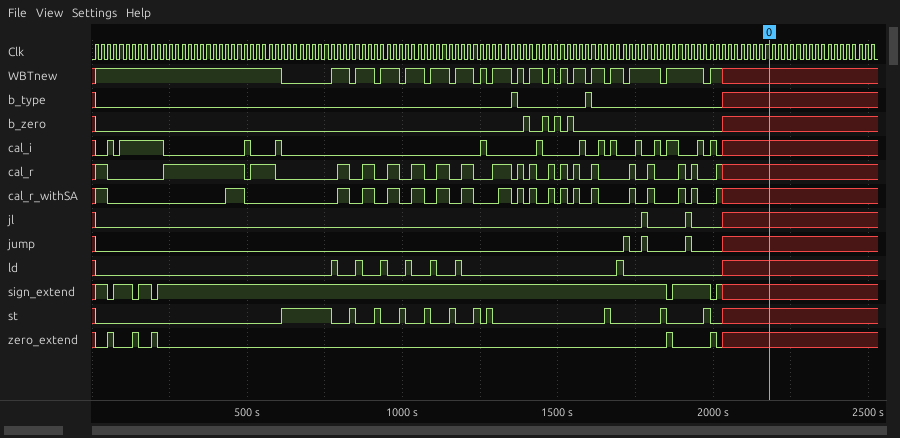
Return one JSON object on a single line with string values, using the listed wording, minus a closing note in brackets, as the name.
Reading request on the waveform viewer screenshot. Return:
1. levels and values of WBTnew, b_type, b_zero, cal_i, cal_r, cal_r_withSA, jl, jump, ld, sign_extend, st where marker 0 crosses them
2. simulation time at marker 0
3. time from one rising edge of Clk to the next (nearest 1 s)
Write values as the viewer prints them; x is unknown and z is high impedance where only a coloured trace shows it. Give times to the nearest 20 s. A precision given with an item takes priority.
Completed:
{"levels and values of WBTnew, b_type, b_zero, cal_i, cal_r, cal_r_withSA, jl, jump, ld, sign_extend, st where marker 0 crosses them": "WBTnew=x, b_type=x, b_zero=x, cal_i=x, cal_r=x, cal_r_withSA=x, jl=x, jump=x, ld=x, sign_extend=x, st=x", "simulation time at marker 0": "2180 s", "time from one rising edge of Clk to the next": "20 s"}
